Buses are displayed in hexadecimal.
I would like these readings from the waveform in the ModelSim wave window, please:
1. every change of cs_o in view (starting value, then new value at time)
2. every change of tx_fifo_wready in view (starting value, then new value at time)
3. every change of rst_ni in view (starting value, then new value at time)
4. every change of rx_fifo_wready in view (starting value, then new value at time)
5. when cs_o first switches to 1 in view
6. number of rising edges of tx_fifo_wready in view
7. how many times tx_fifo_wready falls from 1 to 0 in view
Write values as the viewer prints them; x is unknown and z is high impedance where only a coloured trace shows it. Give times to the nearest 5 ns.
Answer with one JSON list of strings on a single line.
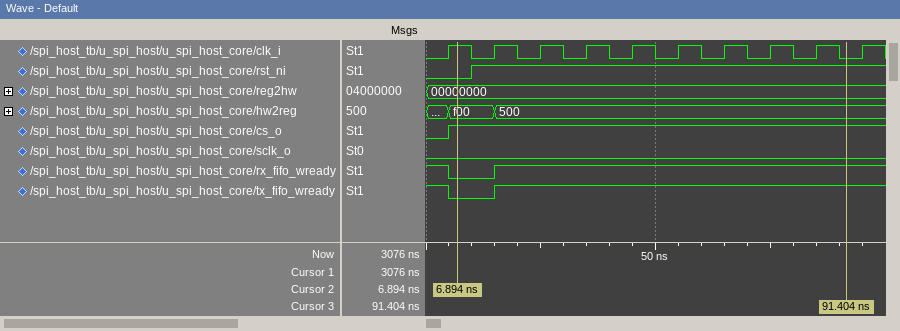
["0, 1 at 5 ns", "1, 0 at 5 ns, 1 at 15 ns", "0, 1 at 10 ns", "1, 0 at 5 ns, 1 at 15 ns", "5 ns", "1", "1"]
